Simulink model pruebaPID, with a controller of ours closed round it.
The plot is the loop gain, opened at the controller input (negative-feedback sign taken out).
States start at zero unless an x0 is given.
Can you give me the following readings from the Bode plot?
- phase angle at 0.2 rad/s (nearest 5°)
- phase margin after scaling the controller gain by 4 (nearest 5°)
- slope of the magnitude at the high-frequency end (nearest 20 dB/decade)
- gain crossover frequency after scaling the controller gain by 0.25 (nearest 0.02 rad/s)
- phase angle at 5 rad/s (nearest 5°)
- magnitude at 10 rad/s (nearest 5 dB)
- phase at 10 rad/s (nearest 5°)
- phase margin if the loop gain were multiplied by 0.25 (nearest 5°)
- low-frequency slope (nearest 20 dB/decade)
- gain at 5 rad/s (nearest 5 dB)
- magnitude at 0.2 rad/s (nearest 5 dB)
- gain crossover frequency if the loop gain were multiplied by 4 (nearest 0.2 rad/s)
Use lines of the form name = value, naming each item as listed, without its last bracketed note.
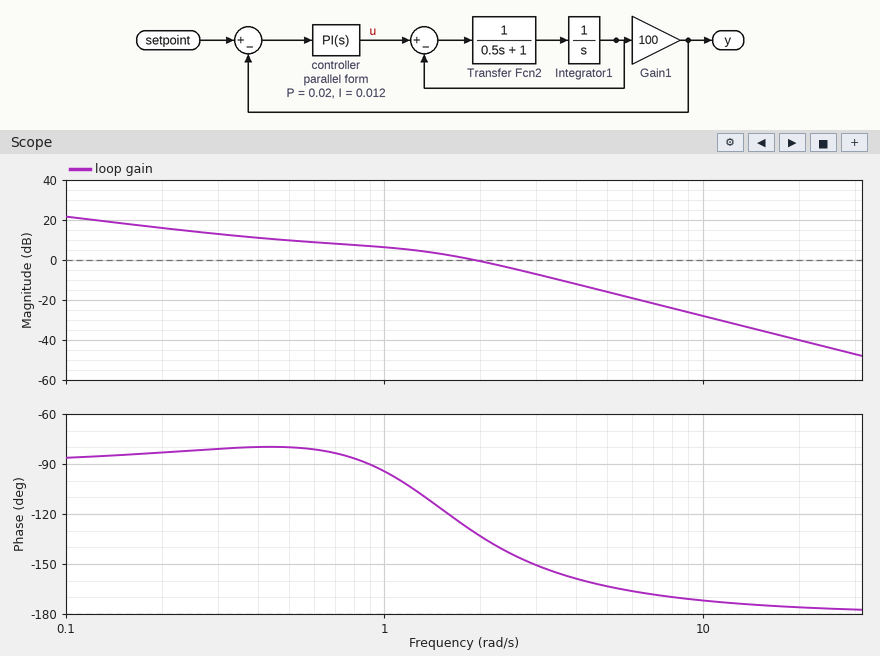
phase angle at 0.2 rad/s = -85°
phase margin after scaling the controller gain by 4 = 20°
slope of the magnitude at the high-frequency end = -40 dB/decade
gain crossover frequency after scaling the controller gain by 0.25 = 0.34 rad/s
phase angle at 5 rad/s = -165°
magnitude at 10 rad/s = -30 dB
phase at 10 rad/s = -170°
phase margin if the loop gain were multiplied by 0.25 = 100°
low-frequency slope = -20 dB/decade
gain at 5 rad/s = -15 dB
magnitude at 0.2 rad/s = 15 dB
gain crossover frequency if the loop gain were multiplied by 4 = 4.0 rad/s
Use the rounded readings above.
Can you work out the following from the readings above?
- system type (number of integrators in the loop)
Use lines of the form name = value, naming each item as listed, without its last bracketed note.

system type = 1
